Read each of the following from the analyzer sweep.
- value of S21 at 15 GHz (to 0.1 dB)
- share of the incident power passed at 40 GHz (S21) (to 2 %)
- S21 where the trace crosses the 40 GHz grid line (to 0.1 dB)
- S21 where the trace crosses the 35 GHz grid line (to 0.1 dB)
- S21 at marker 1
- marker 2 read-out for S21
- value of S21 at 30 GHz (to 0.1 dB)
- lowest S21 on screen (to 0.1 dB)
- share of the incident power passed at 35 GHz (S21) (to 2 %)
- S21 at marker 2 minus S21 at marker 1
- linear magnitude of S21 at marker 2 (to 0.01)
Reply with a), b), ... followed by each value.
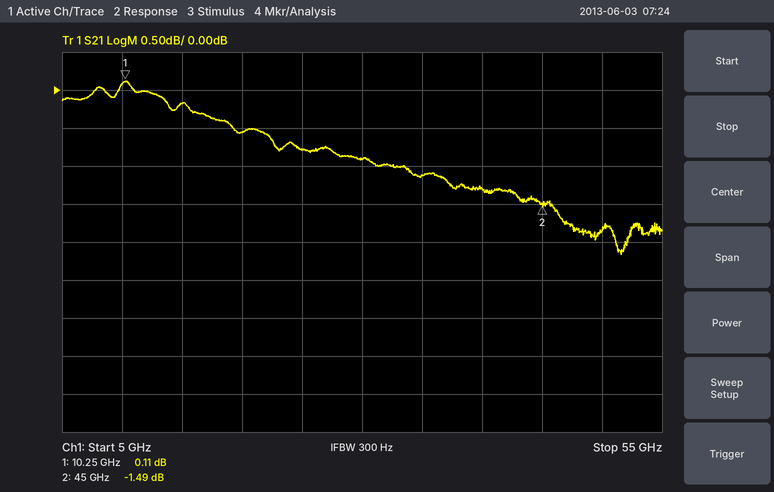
a) -0.2 dB
b) 74 %
c) -1.3 dB
d) -1.1 dB
e) 0.11 dB
f) -1.49 dB
g) -0.9 dB
h) -2.2 dB
i) 78 %
j) -1.60 dB
k) 0.84
